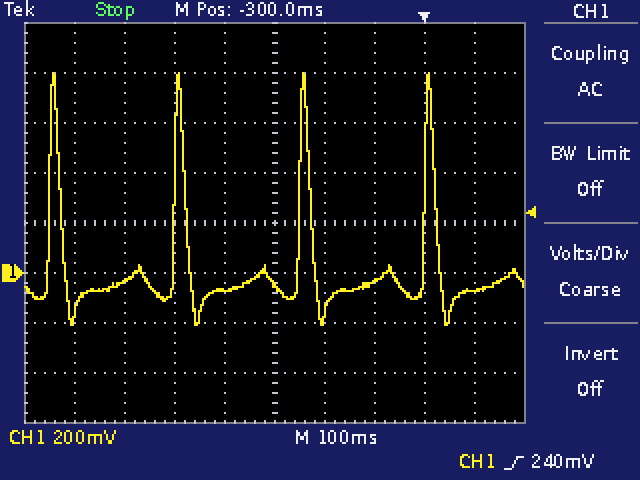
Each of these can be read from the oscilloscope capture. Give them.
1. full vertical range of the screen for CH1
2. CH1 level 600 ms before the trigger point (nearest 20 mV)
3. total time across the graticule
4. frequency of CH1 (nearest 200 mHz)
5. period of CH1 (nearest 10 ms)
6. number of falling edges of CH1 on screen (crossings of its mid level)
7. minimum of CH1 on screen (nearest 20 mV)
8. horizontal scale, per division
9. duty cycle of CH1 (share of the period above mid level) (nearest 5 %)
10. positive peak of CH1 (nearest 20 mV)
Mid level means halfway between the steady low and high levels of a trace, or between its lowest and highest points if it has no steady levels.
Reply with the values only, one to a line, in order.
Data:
1.6 V
-40 mV
1 s
4.0 Hz
250 ms
4
-200 mV
100 ms
10 %
800 mV
